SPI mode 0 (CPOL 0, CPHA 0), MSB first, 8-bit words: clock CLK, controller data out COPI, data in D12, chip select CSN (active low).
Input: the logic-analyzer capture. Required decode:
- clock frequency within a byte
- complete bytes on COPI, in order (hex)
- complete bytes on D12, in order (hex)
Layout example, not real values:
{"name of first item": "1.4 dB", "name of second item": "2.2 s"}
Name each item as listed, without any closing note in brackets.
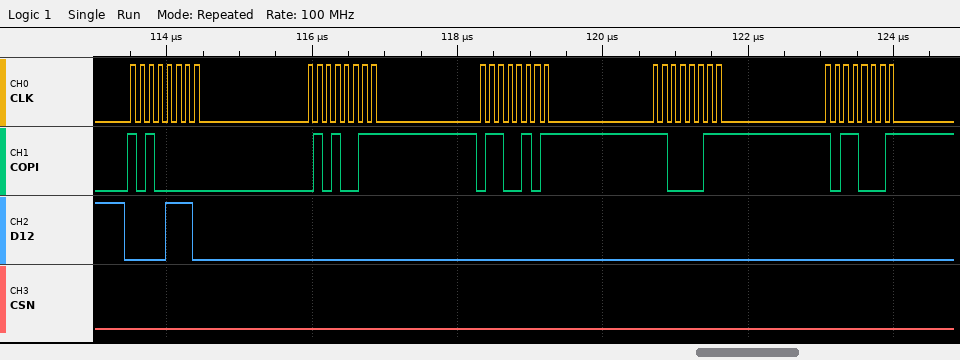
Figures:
{"clock frequency within a byte": "8 MHz", "complete bytes on COPI, in order": "A0 53 65 C3 B1", "complete bytes on D12, in order": "0E 00 00 00 00"}
